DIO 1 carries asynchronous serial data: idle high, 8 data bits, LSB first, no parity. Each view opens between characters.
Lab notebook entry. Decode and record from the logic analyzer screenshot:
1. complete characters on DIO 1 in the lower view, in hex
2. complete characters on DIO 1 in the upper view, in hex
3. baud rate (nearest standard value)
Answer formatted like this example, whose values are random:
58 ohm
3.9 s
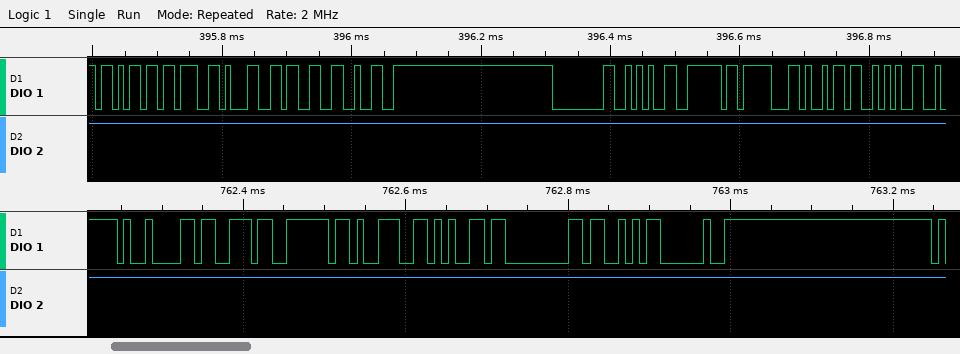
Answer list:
09, 73, 7E, 39, 65, 00, 53, 20
6B, 3B, 31, 33, 32, 00, 2A, 7E, 1F, 69, 2A
115200 baud
